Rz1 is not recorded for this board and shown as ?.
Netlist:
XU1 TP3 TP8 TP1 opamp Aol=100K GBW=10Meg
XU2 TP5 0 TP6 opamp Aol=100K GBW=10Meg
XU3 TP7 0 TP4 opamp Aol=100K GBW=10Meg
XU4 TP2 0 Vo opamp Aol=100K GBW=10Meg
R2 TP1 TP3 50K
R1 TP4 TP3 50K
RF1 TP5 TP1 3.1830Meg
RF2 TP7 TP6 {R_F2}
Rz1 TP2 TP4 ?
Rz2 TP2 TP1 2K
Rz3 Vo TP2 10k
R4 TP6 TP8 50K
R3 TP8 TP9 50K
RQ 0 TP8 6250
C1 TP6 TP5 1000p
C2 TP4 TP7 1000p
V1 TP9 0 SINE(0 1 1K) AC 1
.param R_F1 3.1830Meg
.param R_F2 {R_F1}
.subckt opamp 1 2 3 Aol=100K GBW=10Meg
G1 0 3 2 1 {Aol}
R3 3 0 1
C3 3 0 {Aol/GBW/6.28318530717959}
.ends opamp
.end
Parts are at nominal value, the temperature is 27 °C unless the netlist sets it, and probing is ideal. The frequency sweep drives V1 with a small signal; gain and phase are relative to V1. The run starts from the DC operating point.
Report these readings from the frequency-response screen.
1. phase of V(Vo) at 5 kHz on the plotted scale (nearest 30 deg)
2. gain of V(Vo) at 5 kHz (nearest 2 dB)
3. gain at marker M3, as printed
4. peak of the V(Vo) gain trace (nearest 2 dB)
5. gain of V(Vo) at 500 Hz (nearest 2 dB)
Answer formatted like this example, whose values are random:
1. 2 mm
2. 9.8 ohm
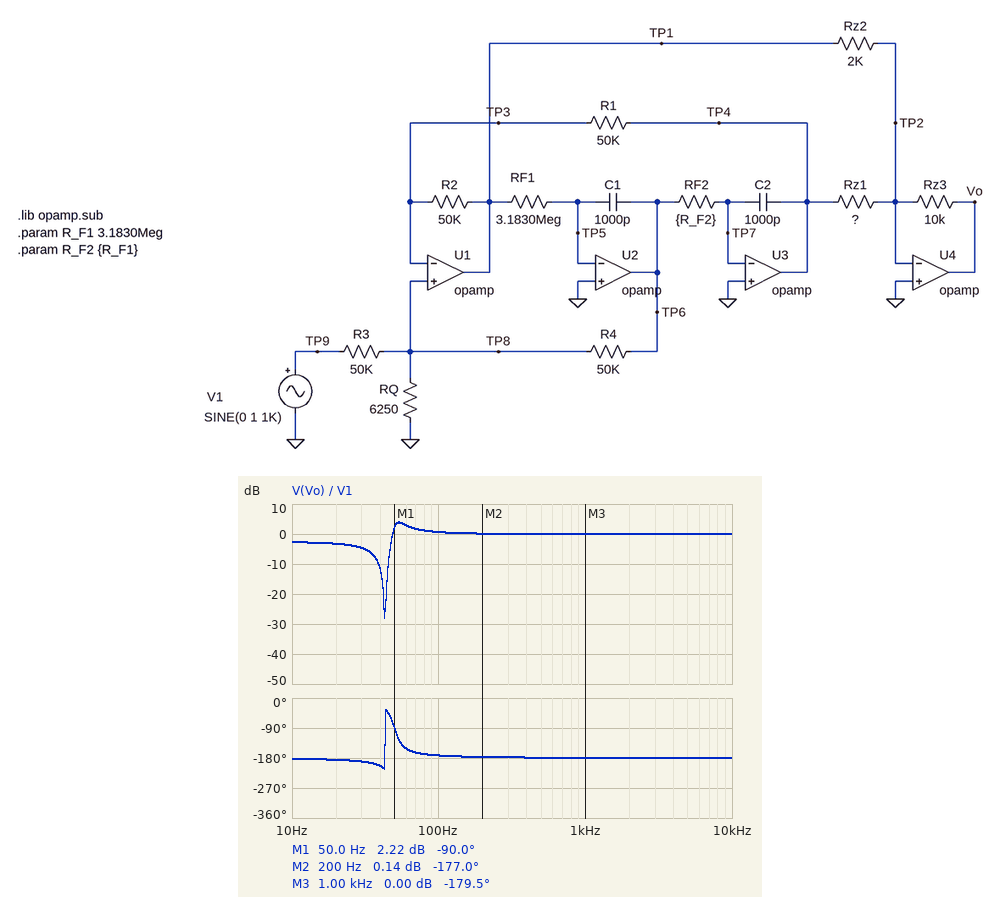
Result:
1. -180 deg
2. 0 dB
3. 0.00 dB
4. 4 dB
5. 0 dB
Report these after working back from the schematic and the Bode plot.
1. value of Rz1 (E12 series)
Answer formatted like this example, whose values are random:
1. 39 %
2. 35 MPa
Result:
1. 2.7 kΩ
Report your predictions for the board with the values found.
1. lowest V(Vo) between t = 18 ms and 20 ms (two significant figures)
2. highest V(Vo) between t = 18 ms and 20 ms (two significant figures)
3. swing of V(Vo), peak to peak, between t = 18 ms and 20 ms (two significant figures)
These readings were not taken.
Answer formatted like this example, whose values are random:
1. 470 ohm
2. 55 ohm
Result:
1. -1.0 V
2. 1.0 V
3. 2.0 V
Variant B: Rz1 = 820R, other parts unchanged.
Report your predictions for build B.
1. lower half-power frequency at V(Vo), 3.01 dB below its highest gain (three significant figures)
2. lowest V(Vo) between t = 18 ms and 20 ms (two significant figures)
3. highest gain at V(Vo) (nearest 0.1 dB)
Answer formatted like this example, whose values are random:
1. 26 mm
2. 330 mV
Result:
1. 42.4 Hz
2. -980 mV
3. 17.4 dB
